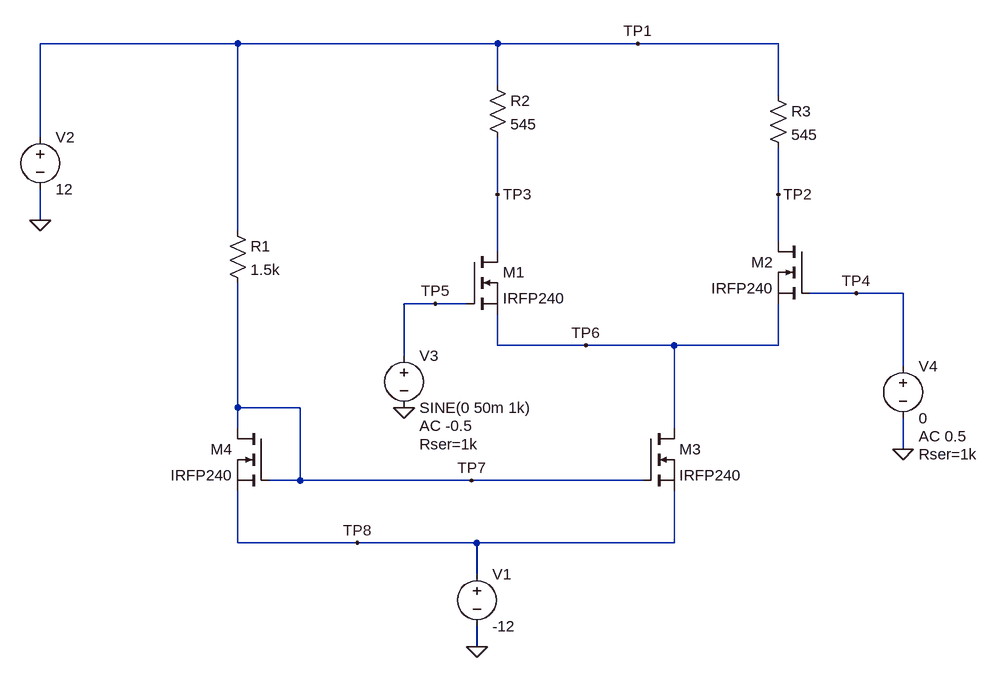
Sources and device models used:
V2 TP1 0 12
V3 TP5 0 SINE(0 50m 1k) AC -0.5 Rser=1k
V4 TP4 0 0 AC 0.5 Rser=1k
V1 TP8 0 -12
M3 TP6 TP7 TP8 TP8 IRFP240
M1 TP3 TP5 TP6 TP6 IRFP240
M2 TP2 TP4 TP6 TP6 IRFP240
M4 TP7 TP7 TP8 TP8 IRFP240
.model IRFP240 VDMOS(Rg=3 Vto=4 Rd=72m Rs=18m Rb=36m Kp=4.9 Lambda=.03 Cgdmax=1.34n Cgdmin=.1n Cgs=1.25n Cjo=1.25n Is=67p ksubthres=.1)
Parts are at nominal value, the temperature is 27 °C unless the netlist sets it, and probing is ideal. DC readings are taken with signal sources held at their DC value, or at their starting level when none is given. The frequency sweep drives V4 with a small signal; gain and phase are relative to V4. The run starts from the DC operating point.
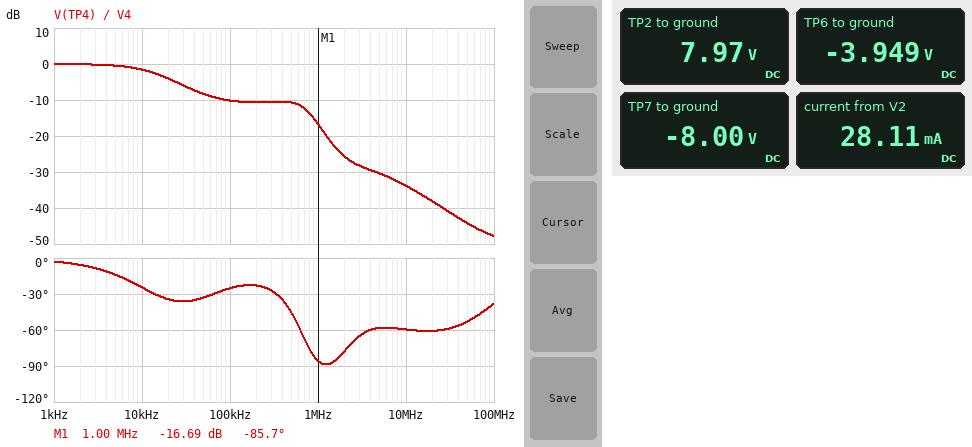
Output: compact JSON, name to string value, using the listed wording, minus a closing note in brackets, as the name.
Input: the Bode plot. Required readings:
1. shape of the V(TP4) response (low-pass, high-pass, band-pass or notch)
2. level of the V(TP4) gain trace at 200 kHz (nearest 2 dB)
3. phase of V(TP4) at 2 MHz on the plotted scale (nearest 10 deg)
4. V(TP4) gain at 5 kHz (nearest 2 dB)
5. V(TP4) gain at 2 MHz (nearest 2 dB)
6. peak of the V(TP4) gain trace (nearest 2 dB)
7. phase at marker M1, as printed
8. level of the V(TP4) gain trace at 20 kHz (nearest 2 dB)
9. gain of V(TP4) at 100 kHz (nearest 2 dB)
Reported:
{"shape of the V(TP4) response": "low-pass", "level of the V(TP4) gain trace at 200 kHz": "-10 dB", "phase of V(TP4) at 2 MHz on the plotted scale": "-80 deg", "V(TP4) gain at 5 kHz": "0 dB", "V(TP4) gain at 2 MHz": "-26 dB", "peak of the V(TP4) gain trace": "0 dB", "phase at marker M1, as printed": "-85.7 deg", "level of the V(TP4) gain trace at 20 kHz": "-4 dB", "gain of V(TP4) at 100 kHz": "-10 dB"}
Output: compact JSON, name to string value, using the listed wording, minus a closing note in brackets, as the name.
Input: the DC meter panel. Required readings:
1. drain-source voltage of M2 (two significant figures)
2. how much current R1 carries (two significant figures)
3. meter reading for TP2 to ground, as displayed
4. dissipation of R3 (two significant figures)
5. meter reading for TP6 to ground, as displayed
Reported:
{"drain-source voltage of M2": "12 V", "how much current R1 carries": "13 mA", "meter reading for TP2 to ground, as displayed": "7.97 V", "dissipation of R3": "30 mW", "meter reading for TP6 to ground, as displayed": "-3.949 V"}
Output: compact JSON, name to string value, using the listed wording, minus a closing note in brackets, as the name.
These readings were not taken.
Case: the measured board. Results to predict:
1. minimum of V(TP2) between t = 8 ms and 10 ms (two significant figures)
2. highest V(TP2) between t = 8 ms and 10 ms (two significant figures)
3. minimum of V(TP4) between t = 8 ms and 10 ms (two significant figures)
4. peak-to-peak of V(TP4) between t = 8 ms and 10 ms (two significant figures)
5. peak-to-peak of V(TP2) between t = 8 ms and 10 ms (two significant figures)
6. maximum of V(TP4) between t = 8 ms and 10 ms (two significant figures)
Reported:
{"minimum of V(TP2) between t = 8 ms and 10 ms": "6.6 V", "highest V(TP2) between t = 8 ms and 10 ms": "9.4 V", "minimum of V(TP4) between t = 8 ms and 10 ms": "-1.7 mV", "peak-to-peak of V(TP4) between t = 8 ms and 10 ms": "3.3 mV", "peak-to-peak of V(TP2) between t = 8 ms and 10 ms": "2.8 V", "maximum of V(TP4) between t = 8 ms and 10 ms": "1.7 mV"}
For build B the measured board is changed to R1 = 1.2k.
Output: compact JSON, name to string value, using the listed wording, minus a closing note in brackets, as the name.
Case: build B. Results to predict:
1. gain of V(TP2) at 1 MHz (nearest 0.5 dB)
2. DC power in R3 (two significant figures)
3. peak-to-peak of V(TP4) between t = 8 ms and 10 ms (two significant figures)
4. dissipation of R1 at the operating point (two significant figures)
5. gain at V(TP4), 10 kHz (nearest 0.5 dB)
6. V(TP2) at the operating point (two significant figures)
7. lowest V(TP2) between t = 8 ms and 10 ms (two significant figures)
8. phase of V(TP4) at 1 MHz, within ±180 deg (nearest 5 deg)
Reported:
{"gain of V(TP2) at 1 MHz": "-3.0 dB", "DC power in R3": "46 mW", "peak-to-peak of V(TP4) between t = 8 ms and 10 ms": "4.1 mV", "dissipation of R1 at the operating point": "330 mW", "gain at V(TP4), 10 kHz": "-2.0 dB", "V(TP2) at the operating point": "7.0 V", "lowest V(TP2) between t = 8 ms and 10 ms": "5.3 V", "phase of V(TP4) at 1 MHz, within ±180 deg": "-85 deg"}
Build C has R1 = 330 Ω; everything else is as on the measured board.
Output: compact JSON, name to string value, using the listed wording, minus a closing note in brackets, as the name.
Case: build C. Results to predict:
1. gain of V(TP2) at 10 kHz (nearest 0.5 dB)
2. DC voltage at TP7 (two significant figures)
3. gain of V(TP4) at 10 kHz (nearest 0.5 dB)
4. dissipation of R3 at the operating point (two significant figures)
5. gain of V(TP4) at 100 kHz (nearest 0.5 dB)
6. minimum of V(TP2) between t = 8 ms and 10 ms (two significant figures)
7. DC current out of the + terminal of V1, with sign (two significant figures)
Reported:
{"gain of V(TP2) at 10 kHz": "-36.5 dB", "DC voltage at TP7": "-7.9 V", "gain of V(TP4) at 10 kHz": "0 dB", "dissipation of R3 at the operating point": "560 mW", "gain of V(TP4) at 100 kHz": "-6.0 dB", "minimum of V(TP2) between t = 8 ms and 10 ms": "-5.5 V", "DC current out of the + terminal of V1, with sign": "-120 mA"}
